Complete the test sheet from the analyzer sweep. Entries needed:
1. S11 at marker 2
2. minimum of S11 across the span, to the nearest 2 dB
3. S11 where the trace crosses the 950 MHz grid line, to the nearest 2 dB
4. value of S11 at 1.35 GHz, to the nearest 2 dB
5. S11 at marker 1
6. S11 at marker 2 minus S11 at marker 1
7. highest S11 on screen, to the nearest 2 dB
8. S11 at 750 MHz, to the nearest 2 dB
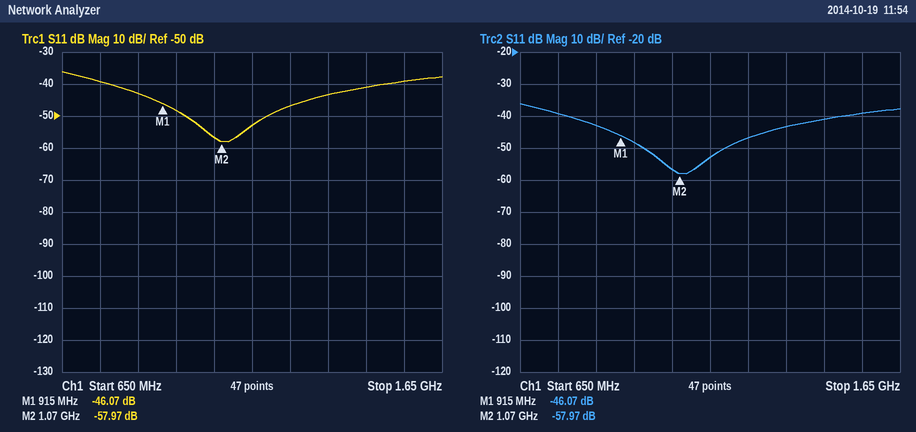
-57.97 dB
-58 dB
-48 dB
-44 dB
-46.07 dB
-11.90 dB
-36 dB
-40 dB
